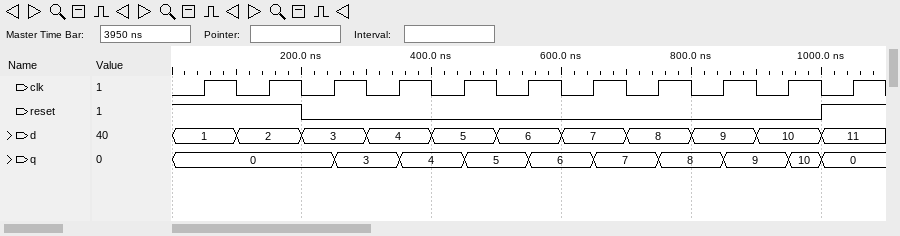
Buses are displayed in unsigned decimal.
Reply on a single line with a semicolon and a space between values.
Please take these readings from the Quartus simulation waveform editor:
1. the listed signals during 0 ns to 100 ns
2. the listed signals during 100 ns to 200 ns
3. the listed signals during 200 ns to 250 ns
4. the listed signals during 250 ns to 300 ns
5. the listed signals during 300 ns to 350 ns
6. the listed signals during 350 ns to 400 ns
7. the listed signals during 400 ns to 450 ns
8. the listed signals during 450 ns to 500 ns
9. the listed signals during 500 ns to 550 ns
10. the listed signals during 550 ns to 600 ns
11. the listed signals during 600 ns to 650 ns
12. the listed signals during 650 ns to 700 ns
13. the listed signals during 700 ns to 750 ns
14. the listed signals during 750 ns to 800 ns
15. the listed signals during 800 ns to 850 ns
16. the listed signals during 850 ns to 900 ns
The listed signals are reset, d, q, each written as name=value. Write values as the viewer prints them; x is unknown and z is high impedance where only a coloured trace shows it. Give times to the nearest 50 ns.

reset=1, d=1, q=0; reset=1, d=2, q=0; reset=0, d=3, q=0; reset=0, d=3, q=3; reset=0, d=4, q=3; reset=0, d=4, q=4; reset=0, d=5, q=4; reset=0, d=5, q=5; reset=0, d=6, q=5; reset=0, d=6, q=6; reset=0, d=7, q=6; reset=0, d=7, q=7; reset=0, d=8, q=7; reset=0, d=8, q=8; reset=0, d=9, q=8; reset=0, d=9, q=9
